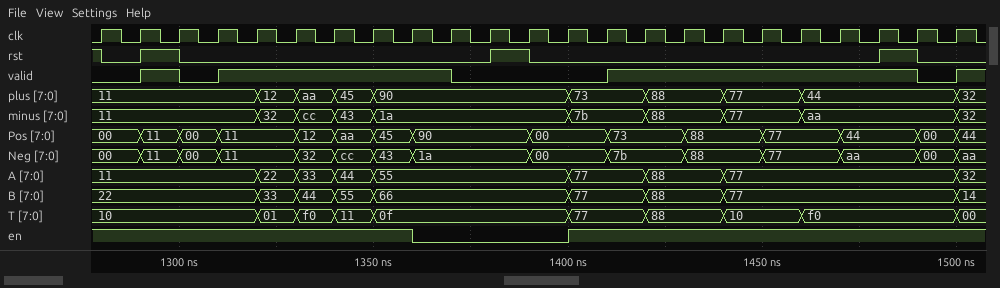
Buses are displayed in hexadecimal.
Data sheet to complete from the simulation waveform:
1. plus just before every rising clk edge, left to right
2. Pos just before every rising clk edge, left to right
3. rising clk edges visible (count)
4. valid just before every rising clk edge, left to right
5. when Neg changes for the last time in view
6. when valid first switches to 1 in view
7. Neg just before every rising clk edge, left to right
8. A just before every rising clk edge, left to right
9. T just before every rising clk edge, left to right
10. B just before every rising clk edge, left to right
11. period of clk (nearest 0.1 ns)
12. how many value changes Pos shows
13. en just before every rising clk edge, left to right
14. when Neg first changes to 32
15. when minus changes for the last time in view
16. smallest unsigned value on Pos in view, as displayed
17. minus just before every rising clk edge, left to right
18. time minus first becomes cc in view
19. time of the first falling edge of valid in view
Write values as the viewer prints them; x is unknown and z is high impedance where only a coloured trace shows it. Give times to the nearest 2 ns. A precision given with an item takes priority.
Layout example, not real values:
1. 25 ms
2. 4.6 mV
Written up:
1. 11, 11, 11, 11, 11, 12, aa, 45, 90, 90, 90, 90, 90, 73, 73, 88, 88, 77, 77, 44, 44, 44, 44
2. 00, 00, 11, 00, 11, 11, 12, aa, 45, 90, 90, 90, 00, 00, 73, 73, 88, 88, 77, 77, 44, 44, 00
3. 23
4. 0 0 1 0 1 1 1 1 1 1 0 0 0 0 1 1 1 1 1 1 1 1 0
5. 1500 ns
6. 1290 ns
7. 00, 00, 11, 00, 11, 11, 32, cc, 43, 1a, 1a, 1a, 00, 00, 7b, 7b, 88, 88, 77, 77, aa, aa, 00
8. 11, 11, 11, 11, 11, 22, 33, 44, 55, 55, 55, 55, 55, 77, 77, 88, 88, 77, 77, 77, 77, 77, 77
9. 10, 10, 10, 10, 10, 01, f0, 11, 0f, 0f, 0f, 0f, 0f, 77, 77, 88, 88, 10, 10, f0, f0, f0, f0
10. 22, 22, 22, 22, 22, 33, 44, 55, 66, 66, 66, 66, 66, 77, 77, 88, 88, 77, 77, 77, 77, 77, 77
11. 10 ns
12. 14
13. 1 1 1 1 1 1 1 1 1 0 0 0 0 1 1 1 1 1 1 1 1 1 1
14. 1330 ns
15. 1500 ns
16. 00
17. 11, 11, 11, 11, 11, 32, cc, 43, 1a, 1a, 1a, 1a, 1a, 7b, 7b, 88, 88, 77, 77, aa, aa, aa, aa
18. 1330 ns
19. 1300 ns
